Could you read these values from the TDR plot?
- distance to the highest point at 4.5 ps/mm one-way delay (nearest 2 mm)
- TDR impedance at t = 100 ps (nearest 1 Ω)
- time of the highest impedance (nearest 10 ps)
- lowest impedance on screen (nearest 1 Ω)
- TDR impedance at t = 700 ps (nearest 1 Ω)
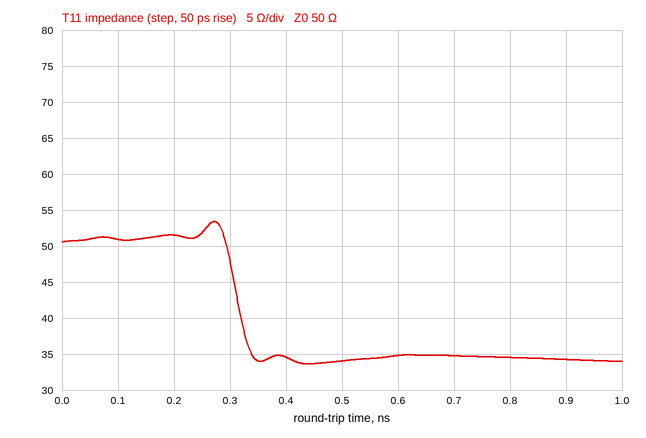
30 mm
51 Ω
270 ps
34 Ω
35 Ω
